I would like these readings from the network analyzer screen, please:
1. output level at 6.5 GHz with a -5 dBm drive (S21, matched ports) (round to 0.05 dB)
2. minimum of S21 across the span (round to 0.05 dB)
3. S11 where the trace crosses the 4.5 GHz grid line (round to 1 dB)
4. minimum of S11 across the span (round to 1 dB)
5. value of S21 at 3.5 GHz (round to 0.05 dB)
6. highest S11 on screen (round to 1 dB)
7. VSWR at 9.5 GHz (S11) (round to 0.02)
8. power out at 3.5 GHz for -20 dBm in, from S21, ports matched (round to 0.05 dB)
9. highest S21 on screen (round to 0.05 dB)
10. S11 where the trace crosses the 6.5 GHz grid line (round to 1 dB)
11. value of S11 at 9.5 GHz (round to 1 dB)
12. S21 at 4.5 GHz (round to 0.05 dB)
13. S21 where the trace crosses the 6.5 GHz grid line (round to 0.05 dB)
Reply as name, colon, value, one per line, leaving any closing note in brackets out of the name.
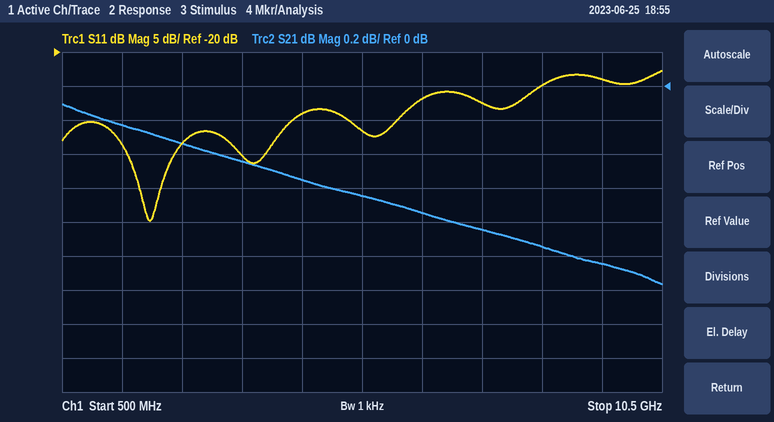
output level at 6.5 GHz with a -5 dBm drive (S21, matched ports): -5.75 dBm
minimum of S21 across the span: -1.15 dB
S11 where the trace crosses the 4.5 GHz grid line: -29 dB
minimum of S11 across the span: -45 dB
value of S21 at 3.5 GHz: -0.45 dB
highest S11 on screen: -23 dB
VSWR at 9.5 GHz (S11): 1.14
power out at 3.5 GHz for -20 dBm in, from S21, ports matched: -20.45 dBm
highest S21 on screen: -0.10 dB
S11 where the trace crosses the 6.5 GHz grid line: -27 dB
value of S11 at 9.5 GHz: -24 dB
S21 at 4.5 GHz: -0.55 dB
S21 where the trace crosses the 6.5 GHz grid line: -0.75 dB
